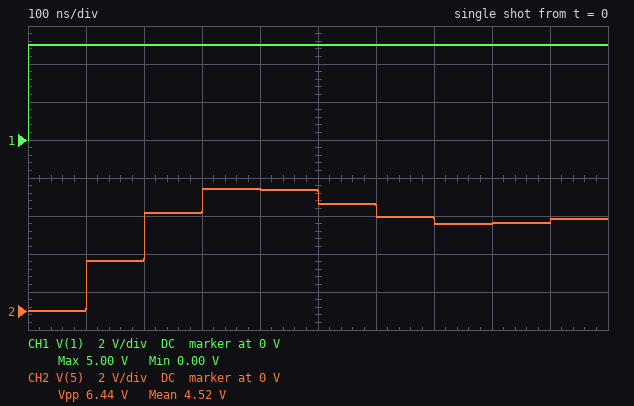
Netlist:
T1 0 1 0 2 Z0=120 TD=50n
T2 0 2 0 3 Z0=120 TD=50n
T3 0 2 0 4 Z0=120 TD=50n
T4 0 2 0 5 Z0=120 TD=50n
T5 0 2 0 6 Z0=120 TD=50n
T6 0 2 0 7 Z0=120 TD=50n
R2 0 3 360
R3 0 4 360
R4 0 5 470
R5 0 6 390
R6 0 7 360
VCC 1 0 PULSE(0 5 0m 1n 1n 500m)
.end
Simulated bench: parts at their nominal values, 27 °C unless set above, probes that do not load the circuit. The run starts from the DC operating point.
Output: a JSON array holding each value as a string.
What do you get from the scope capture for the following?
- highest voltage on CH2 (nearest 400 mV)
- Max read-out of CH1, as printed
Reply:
["6.4 V", "5.00 V"]
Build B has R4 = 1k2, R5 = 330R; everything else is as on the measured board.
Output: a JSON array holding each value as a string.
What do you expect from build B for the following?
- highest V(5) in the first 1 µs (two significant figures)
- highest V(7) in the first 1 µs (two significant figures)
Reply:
["6.7 V", "6.5 V"]
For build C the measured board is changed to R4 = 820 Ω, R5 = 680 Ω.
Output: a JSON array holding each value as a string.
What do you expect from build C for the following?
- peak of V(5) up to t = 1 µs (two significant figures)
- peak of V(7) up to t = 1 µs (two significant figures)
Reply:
["6.9 V", "6.8 V"]
